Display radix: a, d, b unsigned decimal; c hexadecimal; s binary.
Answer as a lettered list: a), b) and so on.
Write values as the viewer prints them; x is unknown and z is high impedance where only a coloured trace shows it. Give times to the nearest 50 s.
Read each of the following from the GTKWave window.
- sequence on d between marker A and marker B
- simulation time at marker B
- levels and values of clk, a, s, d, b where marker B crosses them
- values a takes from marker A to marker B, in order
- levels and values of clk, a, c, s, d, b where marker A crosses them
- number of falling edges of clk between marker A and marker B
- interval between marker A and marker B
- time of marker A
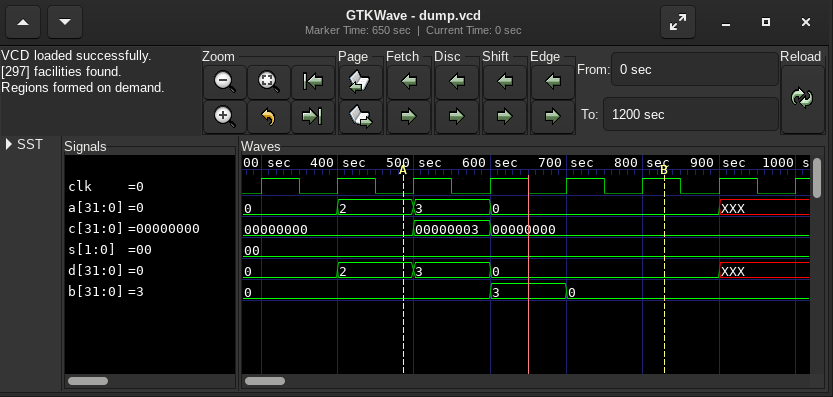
a) 2, 3, 0
b) 850 s
c) clk=1, a=0, s=00, d=0, b=0
d) 2, 3, 0
e) clk=0, a=2, c=00000000, s=00, d=2, b=0
f) 3
g) 350 s
h) 500 s
